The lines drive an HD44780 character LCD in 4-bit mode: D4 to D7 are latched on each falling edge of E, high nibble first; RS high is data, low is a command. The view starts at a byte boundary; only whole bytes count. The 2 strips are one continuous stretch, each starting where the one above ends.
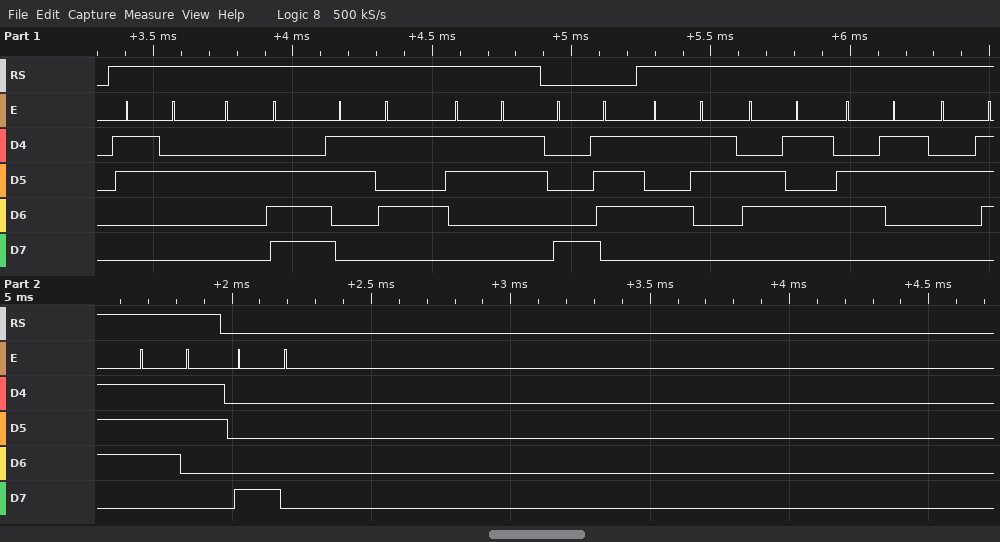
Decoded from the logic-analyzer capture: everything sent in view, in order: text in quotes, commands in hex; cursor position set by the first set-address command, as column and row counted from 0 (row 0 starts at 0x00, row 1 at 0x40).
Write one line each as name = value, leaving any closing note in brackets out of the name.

everything sent in view, in order: text in quotes, commands in hex = "2.53" 0x87 "Sec's" 0x80
cursor position set by the first set-address command, as column and row counted from 0 = column 7, row 0
